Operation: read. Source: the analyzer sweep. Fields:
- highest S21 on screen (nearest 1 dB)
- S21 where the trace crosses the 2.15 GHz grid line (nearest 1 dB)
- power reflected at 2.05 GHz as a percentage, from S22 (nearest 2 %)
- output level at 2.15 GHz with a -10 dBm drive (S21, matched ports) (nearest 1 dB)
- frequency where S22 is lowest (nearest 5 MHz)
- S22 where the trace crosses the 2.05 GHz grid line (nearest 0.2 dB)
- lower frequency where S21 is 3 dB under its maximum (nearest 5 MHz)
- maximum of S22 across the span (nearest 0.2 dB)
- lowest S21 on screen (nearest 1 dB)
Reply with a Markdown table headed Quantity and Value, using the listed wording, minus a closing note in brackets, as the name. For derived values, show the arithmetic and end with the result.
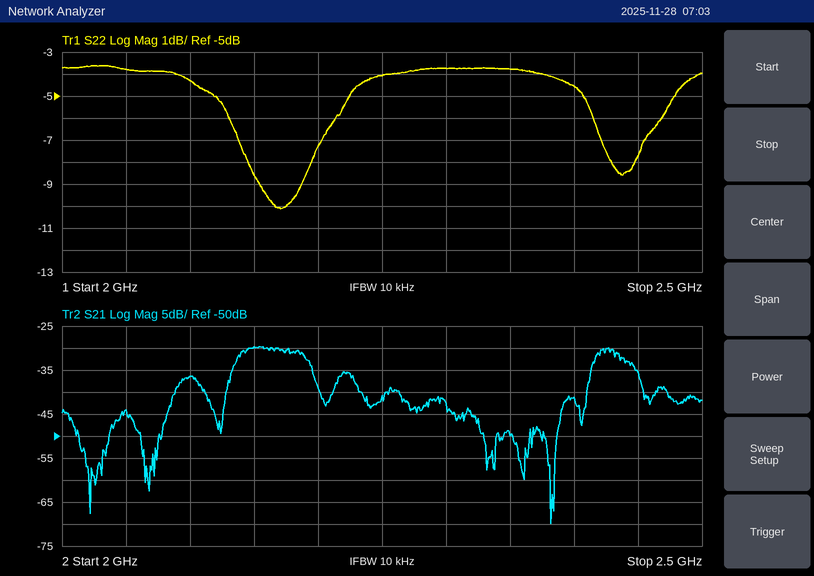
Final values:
| Quantity | Value |
|---|---|
| highest S21 on screen | -30 dB |
| S21 where the trace crosses the 2.15 GHz grid line | -30 dB |
| power reflected at 2.05 GHz as a percentage, from S22 | 10^(-3.8/10) ≈ 42 % |
| output level at 2.15 GHz with a -10 dBm drive (S21, matched ports) | -10 dBm + (-30 dB) = -40 dBm |
| frequency where S22 is lowest | 2.170 GHz |
| S22 where the trace crosses the 2.05 GHz grid line | -3.8 dB |
| lower frequency where S21 is 3 dB under its maximum | 2.135 GHz |
| maximum of S22 across the span | -3.6 dB |
| lowest S21 on screen | -70 dB |
